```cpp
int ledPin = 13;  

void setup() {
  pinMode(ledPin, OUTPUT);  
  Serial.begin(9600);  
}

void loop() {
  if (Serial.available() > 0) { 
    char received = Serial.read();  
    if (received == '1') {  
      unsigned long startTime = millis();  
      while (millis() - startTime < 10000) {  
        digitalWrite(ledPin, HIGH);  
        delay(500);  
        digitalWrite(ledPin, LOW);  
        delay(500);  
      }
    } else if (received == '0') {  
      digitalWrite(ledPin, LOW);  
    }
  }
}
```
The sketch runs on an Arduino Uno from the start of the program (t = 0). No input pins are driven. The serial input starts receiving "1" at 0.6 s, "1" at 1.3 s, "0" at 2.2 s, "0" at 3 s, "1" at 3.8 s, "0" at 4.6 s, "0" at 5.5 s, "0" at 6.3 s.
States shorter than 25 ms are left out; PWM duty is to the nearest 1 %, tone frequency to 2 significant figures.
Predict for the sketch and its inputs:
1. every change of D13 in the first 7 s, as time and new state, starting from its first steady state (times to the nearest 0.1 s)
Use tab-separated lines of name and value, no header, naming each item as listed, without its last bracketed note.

every change of D13 in the first 7 s, as time and new state, starting from its first steady state	0 s low; 0.6 s high; 1.1 s low; 1.6 s high; 2.1 s low; 2.6 s high; 3.1 s low; 3.6 s high; 4.1 s low; 4.6 s high; 5.1 s low; 5.6 s high; 6.1 s low; 6.6 s high
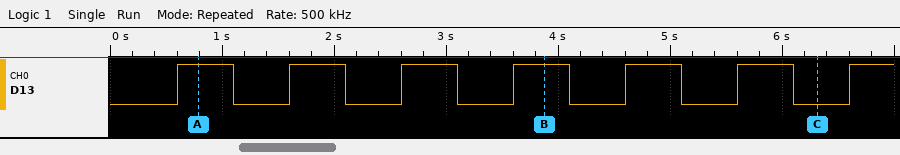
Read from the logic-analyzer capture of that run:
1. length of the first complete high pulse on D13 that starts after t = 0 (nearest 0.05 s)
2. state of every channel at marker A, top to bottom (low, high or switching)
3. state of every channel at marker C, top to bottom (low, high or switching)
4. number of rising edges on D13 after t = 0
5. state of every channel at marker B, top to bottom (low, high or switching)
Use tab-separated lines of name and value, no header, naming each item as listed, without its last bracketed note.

length of the first complete high pulse on D13 that starts after t = 0	0.50 s
state of every channel at marker A, top to bottom	D13 high
state of every channel at marker C, top to bottom	D13 low
number of rising edges on D13 after t = 0	7
state of every channel at marker B, top to bottom	D13 high
